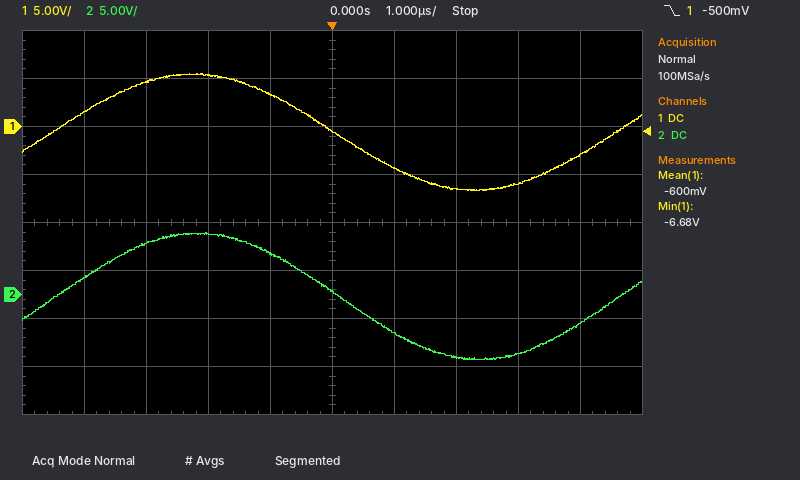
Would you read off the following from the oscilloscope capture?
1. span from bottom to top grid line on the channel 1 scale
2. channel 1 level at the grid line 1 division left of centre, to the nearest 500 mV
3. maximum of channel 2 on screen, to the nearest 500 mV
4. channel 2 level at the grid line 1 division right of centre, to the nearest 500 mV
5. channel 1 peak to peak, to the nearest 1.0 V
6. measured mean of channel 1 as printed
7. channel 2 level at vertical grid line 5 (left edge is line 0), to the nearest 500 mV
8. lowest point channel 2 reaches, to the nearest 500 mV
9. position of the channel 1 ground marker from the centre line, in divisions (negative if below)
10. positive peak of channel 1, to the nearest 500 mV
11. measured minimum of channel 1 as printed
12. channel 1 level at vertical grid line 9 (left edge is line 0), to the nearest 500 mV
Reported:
40 V
3.5 V
6.5 V
-4.0 V
12.0 V
-600 mV
500 mV
-7.0 V
+2.0 div
5.5 V
-6.68 V
-3.0 V
